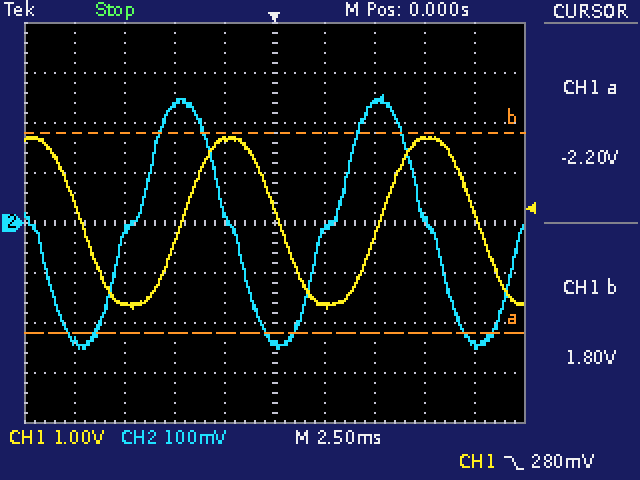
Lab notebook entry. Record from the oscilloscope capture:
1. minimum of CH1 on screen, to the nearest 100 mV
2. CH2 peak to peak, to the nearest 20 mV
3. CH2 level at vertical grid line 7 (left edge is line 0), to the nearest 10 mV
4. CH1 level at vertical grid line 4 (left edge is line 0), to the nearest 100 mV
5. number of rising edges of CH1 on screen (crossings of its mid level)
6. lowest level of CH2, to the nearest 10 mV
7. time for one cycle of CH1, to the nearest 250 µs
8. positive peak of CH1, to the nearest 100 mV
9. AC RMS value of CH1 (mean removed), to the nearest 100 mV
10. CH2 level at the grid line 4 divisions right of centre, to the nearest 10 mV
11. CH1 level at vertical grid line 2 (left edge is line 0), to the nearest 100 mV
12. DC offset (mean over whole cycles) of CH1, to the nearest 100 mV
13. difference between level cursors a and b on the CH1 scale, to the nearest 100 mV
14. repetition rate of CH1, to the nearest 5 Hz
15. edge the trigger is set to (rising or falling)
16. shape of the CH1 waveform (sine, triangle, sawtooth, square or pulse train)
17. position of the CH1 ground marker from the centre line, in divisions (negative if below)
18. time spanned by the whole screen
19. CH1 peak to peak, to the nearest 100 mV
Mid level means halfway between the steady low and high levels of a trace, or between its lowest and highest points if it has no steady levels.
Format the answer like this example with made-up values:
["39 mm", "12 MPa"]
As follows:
["-1.7 V", "500 mV", "240 mV", "1.7 V", "2", "-250 mV", "10.00 ms", "1.7 V", "1.2 V", "-240 mV", "-1.6 V", "0.0 V", "4.0 V", "100 Hz", "falling", "sine", "0.0 div", "25 ms", "3.4 V"]
